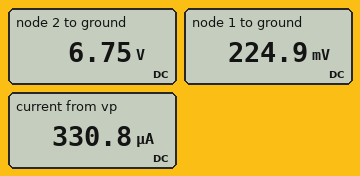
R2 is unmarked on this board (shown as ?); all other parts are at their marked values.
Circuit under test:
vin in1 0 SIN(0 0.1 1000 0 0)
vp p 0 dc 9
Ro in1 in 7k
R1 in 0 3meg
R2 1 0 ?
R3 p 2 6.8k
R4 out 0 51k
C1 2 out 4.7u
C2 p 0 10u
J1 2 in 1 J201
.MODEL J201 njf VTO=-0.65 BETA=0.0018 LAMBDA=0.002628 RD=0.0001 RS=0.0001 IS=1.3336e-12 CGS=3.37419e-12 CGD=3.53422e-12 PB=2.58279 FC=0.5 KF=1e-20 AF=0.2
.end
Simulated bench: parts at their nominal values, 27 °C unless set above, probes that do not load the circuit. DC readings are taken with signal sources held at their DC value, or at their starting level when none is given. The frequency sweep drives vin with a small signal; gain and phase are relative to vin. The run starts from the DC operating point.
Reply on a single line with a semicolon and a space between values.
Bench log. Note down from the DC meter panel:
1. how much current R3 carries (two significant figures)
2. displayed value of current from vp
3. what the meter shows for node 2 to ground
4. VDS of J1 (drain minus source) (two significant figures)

330 µA; 330.8 µA; 6.75 V; 6.5 V
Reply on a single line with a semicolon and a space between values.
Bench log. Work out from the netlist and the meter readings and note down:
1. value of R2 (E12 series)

680 Ω
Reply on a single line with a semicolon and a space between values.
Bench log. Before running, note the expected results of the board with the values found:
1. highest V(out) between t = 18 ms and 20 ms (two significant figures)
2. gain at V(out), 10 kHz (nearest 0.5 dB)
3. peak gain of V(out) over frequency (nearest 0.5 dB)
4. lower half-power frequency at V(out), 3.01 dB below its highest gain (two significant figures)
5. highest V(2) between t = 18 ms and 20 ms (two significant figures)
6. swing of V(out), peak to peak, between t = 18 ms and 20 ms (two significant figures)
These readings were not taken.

440 mV; 13.0 dB; 13.0 dB; 590 mHz; 7.2 V; 900 mV
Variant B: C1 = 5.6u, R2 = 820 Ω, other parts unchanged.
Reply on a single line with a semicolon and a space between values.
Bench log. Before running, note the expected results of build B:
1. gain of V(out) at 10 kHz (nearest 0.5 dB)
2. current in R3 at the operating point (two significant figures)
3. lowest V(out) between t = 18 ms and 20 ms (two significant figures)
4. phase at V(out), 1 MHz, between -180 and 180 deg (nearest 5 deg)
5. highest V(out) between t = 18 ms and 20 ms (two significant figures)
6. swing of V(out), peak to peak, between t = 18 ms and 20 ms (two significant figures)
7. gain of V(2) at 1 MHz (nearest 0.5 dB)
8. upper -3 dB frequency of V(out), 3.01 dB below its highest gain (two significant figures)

12.0 dB; 300 µA; -410 mV; 150 deg; 390 mV; 800 mV; 11.0 dB; 1.9 MHz
